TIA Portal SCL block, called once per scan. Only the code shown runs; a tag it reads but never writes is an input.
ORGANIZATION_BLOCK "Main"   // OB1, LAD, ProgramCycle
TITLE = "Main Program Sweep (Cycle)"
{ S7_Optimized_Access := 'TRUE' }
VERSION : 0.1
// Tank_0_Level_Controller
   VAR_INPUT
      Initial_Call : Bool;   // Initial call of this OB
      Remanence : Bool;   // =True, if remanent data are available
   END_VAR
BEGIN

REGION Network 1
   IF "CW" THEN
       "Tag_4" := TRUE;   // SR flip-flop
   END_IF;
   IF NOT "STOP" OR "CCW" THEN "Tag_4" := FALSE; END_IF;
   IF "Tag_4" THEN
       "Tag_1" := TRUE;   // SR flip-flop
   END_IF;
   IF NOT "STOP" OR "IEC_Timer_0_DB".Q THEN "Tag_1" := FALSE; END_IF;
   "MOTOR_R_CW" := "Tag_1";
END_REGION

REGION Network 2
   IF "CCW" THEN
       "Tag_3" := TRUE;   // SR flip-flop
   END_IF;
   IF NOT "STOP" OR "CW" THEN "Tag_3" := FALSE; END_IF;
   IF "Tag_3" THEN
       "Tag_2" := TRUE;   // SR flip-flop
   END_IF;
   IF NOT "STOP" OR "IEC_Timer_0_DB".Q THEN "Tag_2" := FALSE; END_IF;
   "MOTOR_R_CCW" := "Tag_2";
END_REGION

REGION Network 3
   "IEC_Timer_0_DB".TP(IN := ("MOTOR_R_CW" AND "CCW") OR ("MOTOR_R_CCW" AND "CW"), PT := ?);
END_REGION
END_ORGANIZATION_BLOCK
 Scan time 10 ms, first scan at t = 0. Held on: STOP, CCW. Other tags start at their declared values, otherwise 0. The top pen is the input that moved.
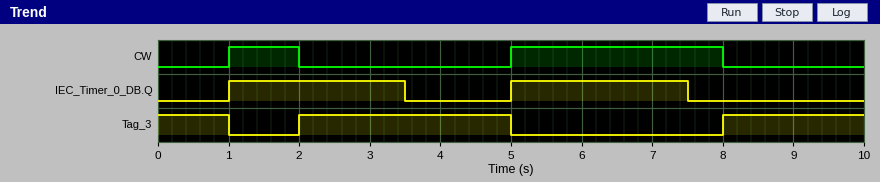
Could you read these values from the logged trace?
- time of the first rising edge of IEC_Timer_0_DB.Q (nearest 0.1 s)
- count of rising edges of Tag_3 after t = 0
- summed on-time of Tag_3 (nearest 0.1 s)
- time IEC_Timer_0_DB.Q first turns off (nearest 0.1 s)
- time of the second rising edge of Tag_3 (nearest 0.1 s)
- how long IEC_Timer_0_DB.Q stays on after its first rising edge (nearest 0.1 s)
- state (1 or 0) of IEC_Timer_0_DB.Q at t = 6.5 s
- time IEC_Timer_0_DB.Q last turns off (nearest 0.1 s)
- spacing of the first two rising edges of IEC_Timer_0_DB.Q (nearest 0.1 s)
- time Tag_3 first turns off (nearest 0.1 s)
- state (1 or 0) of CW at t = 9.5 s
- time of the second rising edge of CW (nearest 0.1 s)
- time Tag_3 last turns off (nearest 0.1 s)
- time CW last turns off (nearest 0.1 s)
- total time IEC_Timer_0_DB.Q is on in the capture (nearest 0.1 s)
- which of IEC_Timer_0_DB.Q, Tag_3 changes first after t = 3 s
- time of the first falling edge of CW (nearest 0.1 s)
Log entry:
1.0 s
2
6.0 s
3.5 s
8.0 s
2.5 s
1
7.5 s
4.0 s
1.0 s
0
5.0 s
5.0 s
8.0 s
5.0 s
IEC_Timer_0_DB.Q
2.0 s
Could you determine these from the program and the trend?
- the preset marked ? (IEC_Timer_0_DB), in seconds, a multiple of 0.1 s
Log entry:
2.5 s
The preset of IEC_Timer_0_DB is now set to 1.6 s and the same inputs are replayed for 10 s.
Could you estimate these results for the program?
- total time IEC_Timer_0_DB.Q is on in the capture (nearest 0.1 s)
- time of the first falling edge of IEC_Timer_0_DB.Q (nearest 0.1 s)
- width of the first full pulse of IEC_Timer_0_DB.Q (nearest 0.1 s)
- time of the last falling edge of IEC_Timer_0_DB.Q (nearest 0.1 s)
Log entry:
3.2 s
2.6 s
1.6 s
6.6 s
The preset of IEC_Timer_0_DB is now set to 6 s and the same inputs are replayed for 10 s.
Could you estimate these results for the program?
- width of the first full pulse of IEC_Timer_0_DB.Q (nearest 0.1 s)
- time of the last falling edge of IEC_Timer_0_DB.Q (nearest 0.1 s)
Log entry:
6.0 s
7.0 s
